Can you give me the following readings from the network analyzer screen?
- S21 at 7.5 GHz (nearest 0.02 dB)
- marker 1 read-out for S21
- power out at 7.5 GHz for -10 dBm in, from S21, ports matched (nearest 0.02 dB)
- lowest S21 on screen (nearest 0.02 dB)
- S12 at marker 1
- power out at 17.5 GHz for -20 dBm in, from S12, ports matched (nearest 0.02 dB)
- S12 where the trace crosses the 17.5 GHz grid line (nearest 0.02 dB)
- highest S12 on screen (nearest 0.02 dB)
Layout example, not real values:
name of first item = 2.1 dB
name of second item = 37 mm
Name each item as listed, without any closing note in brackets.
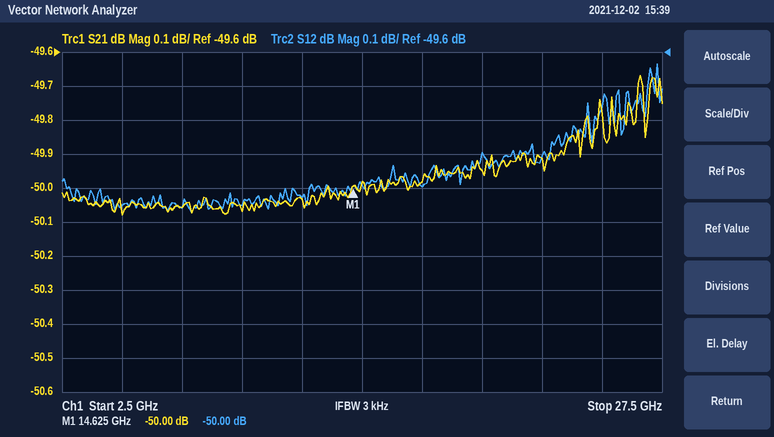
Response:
S21 at 7.5 GHz = -50.06 dB
marker 1 read-out for S21 = -50.00 dB
power out at 7.5 GHz for -10 dBm in, from S21, ports matched = -60.06 dBm
lowest S21 on screen = -50.08 dB
S12 at marker 1 = -50.00 dB
power out at 17.5 GHz for -20 dBm in, from S12, ports matched = -70.00 dBm
S12 where the trace crosses the 17.5 GHz grid line = -50.00 dB
highest S12 on screen = -49.64 dB
